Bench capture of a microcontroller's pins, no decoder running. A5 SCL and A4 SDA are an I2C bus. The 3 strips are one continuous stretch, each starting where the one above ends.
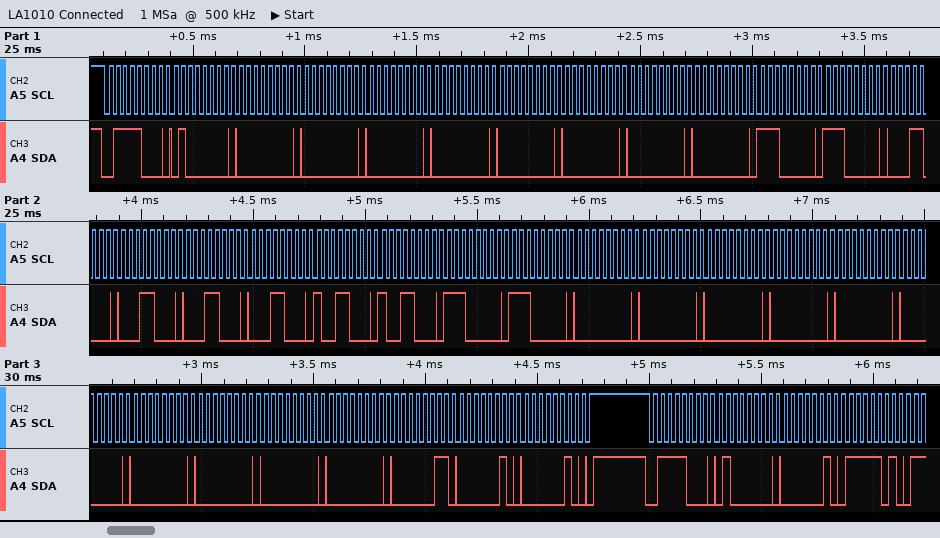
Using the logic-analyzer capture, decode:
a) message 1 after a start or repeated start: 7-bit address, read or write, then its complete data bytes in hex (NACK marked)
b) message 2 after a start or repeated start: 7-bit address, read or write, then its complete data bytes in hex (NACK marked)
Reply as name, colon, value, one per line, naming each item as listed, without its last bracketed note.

message 1 after a start or repeated start: 7-bit address, read or write, then its complete data bytes in hex: 0x3C write: 40 00 00 00 00 00 00 00 00 E0 E0 18 18 18 18 98 98 E0 E0 00 00 00 00 00 00 00 00 00 00 03 02 02
message 2 after a start or repeated start: 7-bit address, read or write, then its complete data bytes in hex: 0x3C write: 40 02 FA
